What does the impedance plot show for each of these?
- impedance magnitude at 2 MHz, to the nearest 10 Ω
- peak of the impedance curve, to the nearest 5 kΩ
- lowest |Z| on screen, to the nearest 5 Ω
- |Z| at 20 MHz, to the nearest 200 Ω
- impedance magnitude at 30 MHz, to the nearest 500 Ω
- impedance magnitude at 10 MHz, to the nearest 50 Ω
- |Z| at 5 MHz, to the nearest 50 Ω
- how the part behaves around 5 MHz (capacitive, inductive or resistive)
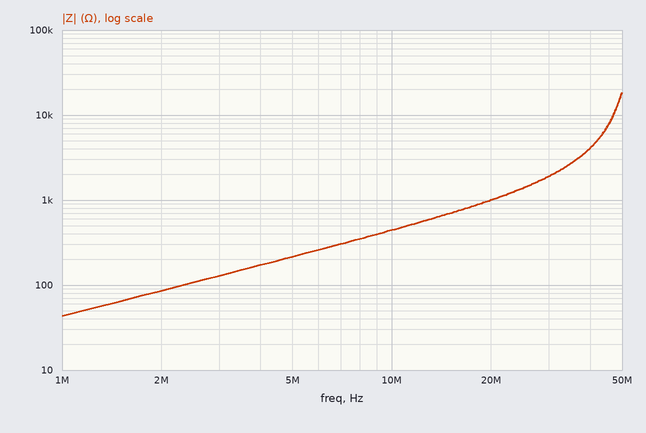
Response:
90 Ω
20 kΩ
45 Ω
1.0 kΩ
2.0 kΩ
450 Ω
200 Ω
inductive
